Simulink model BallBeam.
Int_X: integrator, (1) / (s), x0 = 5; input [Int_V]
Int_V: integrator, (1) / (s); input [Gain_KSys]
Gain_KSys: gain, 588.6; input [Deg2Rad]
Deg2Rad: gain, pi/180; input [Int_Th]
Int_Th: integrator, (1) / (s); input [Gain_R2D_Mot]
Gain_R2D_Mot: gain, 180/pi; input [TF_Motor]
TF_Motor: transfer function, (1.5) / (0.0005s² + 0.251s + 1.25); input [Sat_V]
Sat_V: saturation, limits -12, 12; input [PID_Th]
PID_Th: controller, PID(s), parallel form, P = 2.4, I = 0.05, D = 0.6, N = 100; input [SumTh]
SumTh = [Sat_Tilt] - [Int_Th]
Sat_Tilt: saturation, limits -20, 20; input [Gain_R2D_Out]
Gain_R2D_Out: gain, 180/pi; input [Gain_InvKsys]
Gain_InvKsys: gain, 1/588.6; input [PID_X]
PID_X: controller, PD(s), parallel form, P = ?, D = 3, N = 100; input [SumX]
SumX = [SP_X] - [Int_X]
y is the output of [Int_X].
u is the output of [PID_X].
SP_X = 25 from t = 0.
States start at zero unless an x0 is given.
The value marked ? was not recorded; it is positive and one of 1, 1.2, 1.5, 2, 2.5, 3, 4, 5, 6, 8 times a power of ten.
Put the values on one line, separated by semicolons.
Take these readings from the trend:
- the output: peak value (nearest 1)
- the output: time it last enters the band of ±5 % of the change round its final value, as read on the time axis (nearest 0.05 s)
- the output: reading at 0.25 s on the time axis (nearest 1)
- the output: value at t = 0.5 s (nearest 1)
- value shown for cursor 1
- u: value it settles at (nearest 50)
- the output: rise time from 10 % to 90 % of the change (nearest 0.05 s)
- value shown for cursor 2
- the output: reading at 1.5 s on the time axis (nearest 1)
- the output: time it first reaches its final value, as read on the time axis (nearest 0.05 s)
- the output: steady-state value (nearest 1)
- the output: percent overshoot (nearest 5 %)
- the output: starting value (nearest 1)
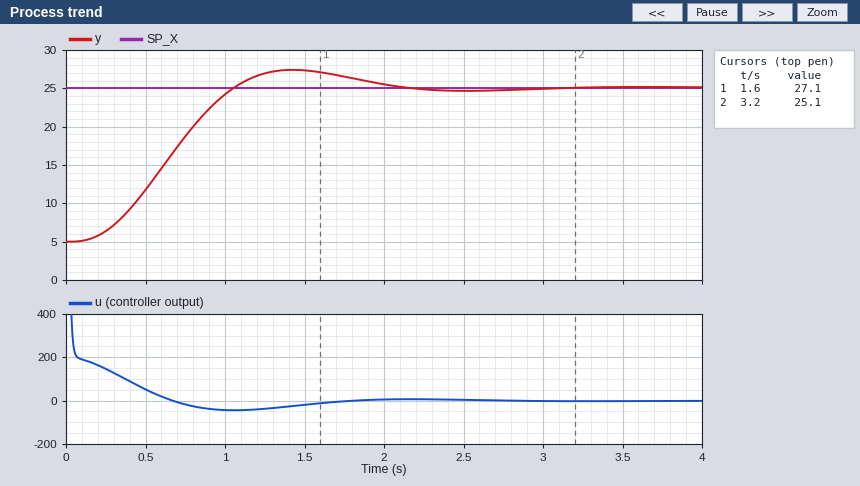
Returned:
27; 1.85 s; 6; 12; 27.1; 0; 0.65 s; 25.1; 27; 1.05 s; 25; 10 %; 5
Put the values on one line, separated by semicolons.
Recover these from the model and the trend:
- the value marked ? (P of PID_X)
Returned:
10
